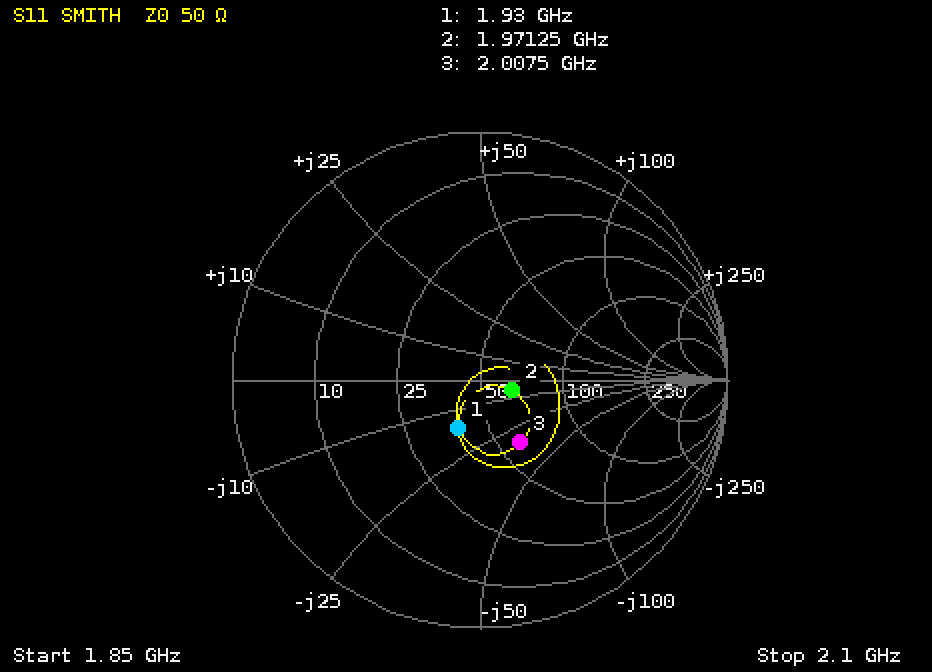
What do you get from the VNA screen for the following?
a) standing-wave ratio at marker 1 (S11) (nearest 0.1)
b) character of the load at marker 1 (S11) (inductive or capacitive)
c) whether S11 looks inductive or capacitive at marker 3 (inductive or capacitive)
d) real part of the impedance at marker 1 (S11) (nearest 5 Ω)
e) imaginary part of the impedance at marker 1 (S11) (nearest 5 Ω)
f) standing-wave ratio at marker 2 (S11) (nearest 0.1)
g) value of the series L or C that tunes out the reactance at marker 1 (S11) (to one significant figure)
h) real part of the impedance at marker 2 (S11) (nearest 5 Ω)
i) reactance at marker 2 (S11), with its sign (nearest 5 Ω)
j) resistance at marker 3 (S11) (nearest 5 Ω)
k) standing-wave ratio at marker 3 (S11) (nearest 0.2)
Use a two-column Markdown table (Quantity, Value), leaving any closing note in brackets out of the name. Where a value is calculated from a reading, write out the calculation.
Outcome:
| Quantity | Value |
|---|---|
| standing-wave ratio at marker 1 (S11) | 1.5 |
| character of the load at marker 1 (S11) | capacitive |
| whether S11 looks inductive or capacitive at marker 3 | capacitive |
| real part of the impedance at marker 1 (S11) | 40 Ω |
| imaginary part of the impedance at marker 1 (S11) | -15 Ω |
| standing-wave ratio at marker 2 (S11) | 1.3 |
| value of the series L or C that tunes out the reactance at marker 1 (S11) | L = 15 Ω/(2π × 1.93 GHz) ≈ 1 nH |
| real part of the impedance at marker 2 (S11) | 65 Ω |
| reactance at marker 2 (S11), with its sign | -5 Ω |
| resistance at marker 3 (S11) | 60 Ω |
| standing-wave ratio at marker 3 (S11) | 1.8 |
